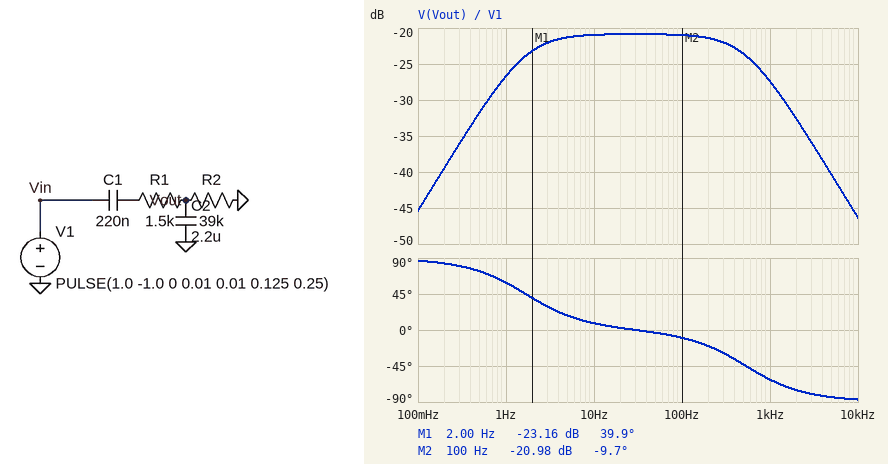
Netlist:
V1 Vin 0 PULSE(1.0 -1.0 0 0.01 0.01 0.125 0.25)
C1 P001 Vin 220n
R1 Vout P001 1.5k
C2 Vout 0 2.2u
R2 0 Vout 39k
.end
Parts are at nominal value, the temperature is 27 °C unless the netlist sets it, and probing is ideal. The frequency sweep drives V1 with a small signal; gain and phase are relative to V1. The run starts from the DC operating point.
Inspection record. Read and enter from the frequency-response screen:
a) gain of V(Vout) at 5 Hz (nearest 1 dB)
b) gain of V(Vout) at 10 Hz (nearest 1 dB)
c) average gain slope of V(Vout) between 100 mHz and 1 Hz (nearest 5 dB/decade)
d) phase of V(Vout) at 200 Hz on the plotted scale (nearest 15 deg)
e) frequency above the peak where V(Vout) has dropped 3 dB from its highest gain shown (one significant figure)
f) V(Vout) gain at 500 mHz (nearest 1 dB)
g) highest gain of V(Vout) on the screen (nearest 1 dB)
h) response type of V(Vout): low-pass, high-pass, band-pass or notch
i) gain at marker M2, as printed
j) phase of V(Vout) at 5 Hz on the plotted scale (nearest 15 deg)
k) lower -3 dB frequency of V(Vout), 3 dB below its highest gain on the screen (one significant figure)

-21 dB
-21 dB
20 dB/decade
-15 deg
500 Hz
-32 dB
-21 dB
band-pass
-20.98 dB
15 deg
2 Hz
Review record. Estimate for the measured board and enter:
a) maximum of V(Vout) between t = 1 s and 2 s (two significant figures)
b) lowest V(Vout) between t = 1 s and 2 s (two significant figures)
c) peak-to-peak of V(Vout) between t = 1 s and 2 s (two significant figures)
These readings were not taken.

140 mV
-130 mV
270 mV
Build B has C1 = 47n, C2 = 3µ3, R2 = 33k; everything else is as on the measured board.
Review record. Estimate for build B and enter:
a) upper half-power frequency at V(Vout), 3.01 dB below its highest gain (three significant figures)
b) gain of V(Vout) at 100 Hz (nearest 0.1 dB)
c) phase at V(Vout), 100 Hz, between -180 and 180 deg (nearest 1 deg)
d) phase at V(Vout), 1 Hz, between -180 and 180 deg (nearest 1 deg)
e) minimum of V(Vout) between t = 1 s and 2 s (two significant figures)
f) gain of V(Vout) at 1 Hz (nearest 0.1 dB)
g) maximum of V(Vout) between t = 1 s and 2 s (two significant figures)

2.29 kHz
-37.1 dB
-2 deg
55 deg
-19 mV
-41.9 dB
21 mV
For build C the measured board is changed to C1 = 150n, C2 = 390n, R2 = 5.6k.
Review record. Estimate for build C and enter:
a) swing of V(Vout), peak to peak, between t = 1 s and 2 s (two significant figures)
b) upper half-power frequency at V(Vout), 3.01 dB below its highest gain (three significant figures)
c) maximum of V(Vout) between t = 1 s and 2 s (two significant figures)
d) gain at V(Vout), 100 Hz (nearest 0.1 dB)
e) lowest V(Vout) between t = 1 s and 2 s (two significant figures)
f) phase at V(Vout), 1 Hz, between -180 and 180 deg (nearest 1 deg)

320 mV
1.10 kHz
160 mV
-12.4 dB
-160 mV
89 deg
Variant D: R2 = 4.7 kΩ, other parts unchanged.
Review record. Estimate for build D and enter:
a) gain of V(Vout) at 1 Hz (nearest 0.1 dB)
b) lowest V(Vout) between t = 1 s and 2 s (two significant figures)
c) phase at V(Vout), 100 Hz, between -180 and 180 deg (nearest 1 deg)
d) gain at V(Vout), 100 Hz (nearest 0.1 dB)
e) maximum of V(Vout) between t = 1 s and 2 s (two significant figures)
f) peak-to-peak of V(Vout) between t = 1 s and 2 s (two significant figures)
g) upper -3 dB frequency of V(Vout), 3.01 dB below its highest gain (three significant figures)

-43.8 dB
-120 mV
-3 deg
-21.1 dB
120 mV
240 mV
559 Hz
